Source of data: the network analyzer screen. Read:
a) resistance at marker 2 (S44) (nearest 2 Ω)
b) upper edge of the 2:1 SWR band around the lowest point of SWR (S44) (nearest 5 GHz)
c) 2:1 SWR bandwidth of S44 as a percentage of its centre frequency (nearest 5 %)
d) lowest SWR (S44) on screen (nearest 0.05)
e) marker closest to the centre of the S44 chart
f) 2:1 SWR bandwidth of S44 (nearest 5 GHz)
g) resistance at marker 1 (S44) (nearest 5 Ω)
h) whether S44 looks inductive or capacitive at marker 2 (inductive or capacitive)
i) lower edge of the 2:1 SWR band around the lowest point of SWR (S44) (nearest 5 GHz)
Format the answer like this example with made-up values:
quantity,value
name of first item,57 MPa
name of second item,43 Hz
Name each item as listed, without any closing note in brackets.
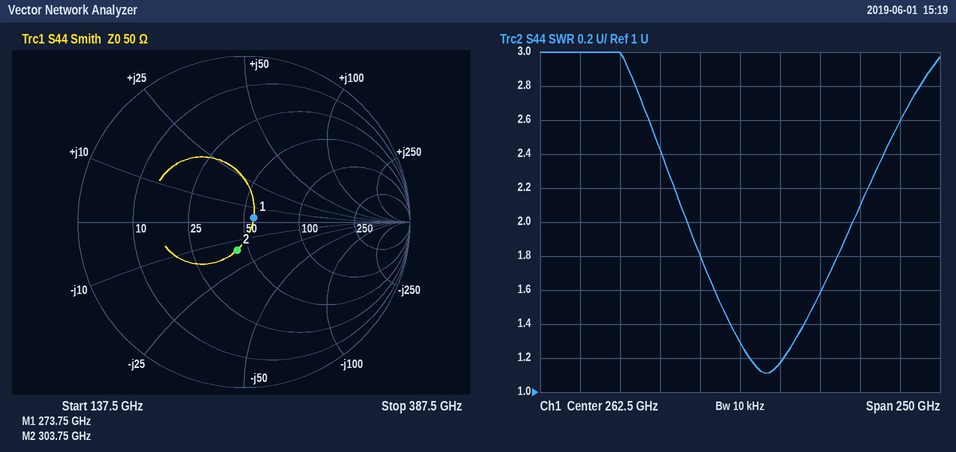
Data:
quantity,value
resistance at marker 2 (S44),44 Ω
upper edge of the 2:1 SWR band around the lowest point of SWR (S44),335 GHz
2:1 SWR bandwidth of S44 as a percentage of its centre frequency,35 %
lowest SWR (S44) on screen,1.10
marker closest to the centre of the S44 chart,marker 1
2:1 SWR bandwidth of S44,105 GHz
resistance at marker 1 (S44),55 Ω
whether S44 looks inductive or capacitive at marker 2,capacitive
lower edge of the 2:1 SWR band around the lowest point of SWR (S44),230 GHz
